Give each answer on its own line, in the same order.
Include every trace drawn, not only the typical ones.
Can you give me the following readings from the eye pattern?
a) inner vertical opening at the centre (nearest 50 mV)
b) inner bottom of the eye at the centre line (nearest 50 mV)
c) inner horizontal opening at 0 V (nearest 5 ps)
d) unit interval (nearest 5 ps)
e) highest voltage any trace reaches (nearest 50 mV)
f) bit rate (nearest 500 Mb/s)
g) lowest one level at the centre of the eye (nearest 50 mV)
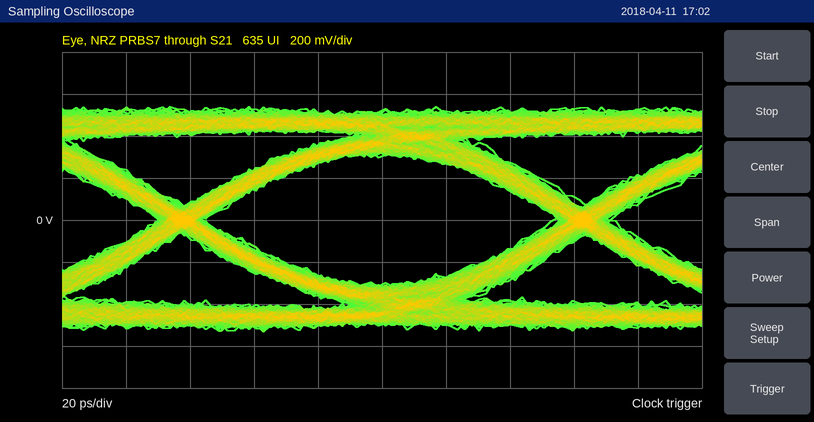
600 mV
-300 mV
110 ps
125 ps
550 mV
8.0 Gb/s
300 mV
